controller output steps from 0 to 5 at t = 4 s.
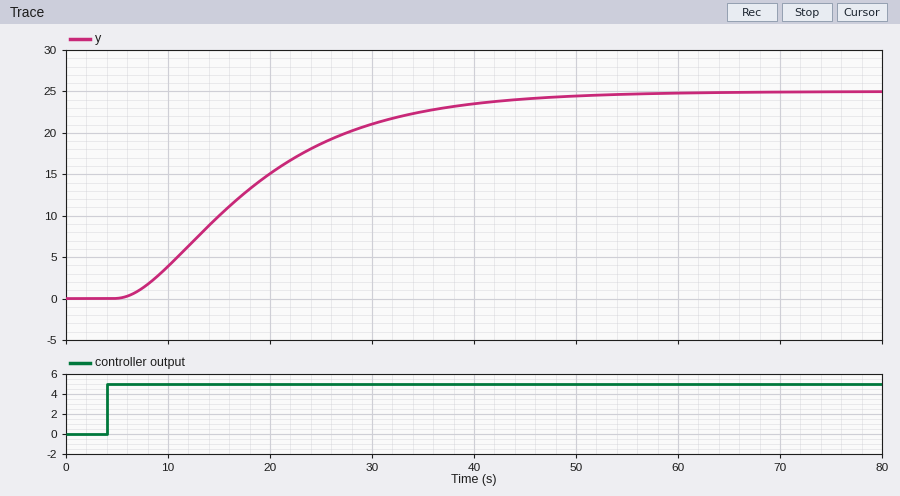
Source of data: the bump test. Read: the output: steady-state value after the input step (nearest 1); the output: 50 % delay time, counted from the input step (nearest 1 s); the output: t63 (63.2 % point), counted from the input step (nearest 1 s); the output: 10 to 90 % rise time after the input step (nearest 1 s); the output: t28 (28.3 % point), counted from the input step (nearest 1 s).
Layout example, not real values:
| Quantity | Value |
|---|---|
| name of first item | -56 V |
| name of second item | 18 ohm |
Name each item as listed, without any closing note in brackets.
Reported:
| Quantity | Value |
|---|---|
| the output: steady-state value after the input step | 25 |
| the output: 50 % delay time, counted from the input step | 13 s |
| the output: t63 (63.2 % point), counted from the input step | 17 s |
| the output: 10 to 90 % rise time after the input step | 26 s |
| the output: t28 (28.3 % point), counted from the input step | 9 s |
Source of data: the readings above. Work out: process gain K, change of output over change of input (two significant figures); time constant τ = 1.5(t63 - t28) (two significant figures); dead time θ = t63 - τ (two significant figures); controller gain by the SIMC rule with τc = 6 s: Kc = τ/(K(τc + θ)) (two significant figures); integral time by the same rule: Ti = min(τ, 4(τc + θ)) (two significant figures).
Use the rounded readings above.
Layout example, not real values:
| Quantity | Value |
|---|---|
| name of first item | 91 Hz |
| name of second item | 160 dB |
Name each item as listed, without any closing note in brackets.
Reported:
| Quantity | Value |
|---|---|
| process gain K, change of output over change of input | 5.0 |
| time constant τ = 1.5(t63 - t28) | 12 s |
| dead time θ = t63 - τ | 5.0 s |
| controller gain by the SIMC rule with τc = 6 s: Kc = τ/(K(τc + θ)) | 0.22 |
| integral time by the same rule: Ti = min(τ, 4(τc + θ)) | 12 s |
